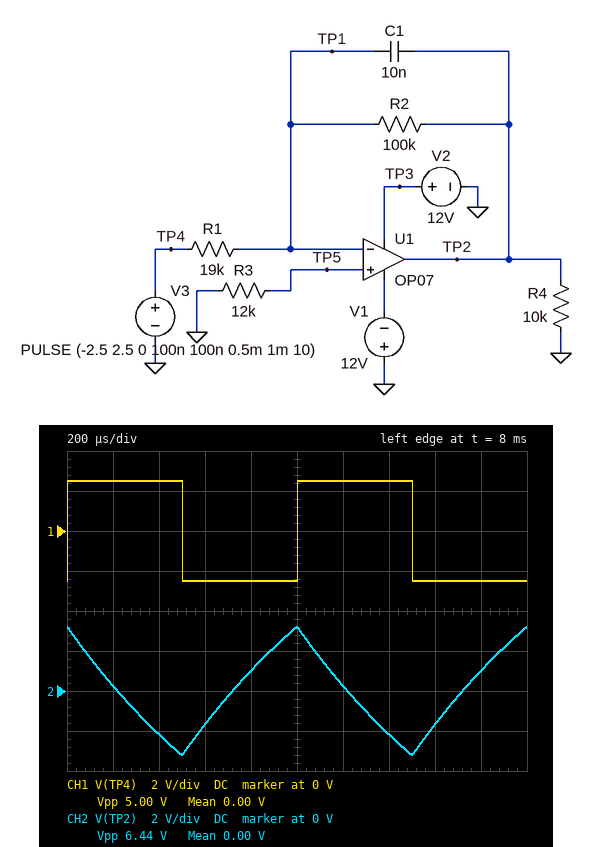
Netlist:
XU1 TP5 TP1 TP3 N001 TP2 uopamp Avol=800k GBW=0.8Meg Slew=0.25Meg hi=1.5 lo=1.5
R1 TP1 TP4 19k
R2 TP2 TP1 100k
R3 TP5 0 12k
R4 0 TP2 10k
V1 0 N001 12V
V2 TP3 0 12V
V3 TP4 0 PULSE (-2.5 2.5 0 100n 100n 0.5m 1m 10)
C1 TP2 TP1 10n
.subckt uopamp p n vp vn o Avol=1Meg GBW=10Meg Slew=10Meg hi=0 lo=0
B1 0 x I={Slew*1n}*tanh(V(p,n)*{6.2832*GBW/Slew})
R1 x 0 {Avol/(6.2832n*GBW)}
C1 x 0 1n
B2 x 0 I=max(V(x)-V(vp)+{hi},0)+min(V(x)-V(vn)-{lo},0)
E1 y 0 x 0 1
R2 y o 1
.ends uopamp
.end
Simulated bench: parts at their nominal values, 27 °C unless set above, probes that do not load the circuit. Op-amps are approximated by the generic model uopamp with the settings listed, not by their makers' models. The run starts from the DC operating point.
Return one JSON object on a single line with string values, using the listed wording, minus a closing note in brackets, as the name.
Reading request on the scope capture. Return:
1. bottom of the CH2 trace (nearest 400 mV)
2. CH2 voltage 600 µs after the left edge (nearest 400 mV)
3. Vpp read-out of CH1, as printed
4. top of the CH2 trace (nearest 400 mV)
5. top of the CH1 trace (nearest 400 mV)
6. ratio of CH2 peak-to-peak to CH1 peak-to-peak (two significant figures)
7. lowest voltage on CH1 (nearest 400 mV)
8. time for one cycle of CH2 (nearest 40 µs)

{"bottom of the CH2 trace": "-3.2 V", "CH2 voltage 600 µs after the left edge": "-1.6 V", "Vpp read-out of CH1, as printed": "5.00 V", "top of the CH2 trace": "3.2 V", "top of the CH1 trace": "2.4 V", "ratio of CH2 peak-to-peak to CH1 peak-to-peak": "1.3", "lowest voltage on CH1": "-2.4 V", "time for one cycle of CH2": "1.00 ms"}
